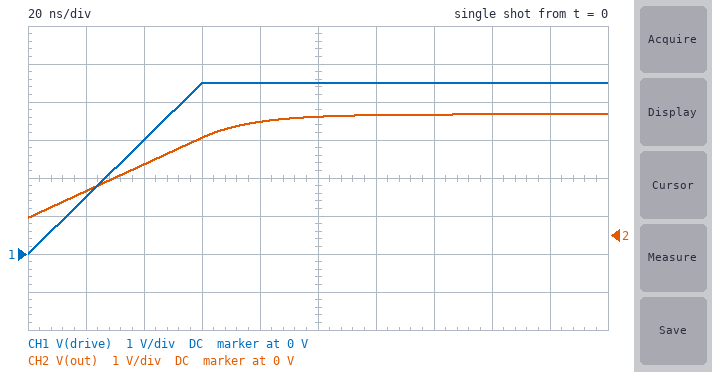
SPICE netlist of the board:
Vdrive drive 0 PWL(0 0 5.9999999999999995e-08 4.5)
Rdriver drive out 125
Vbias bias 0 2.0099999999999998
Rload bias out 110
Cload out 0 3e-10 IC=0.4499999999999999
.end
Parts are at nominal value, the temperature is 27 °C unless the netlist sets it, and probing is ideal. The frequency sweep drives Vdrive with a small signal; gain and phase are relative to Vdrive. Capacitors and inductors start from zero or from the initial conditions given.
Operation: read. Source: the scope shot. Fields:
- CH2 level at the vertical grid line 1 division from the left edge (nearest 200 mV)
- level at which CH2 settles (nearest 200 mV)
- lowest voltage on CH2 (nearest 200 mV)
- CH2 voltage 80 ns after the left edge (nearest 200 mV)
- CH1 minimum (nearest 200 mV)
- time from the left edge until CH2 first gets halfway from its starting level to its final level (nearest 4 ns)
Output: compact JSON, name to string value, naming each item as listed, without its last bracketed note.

{"CH2 level at the vertical grid line 1 division from the left edge": "1.2 V", "level at which CH2 settles": "3.2 V", "lowest voltage on CH2": "400 mV", "CH2 voltage 80 ns after the left edge": "3.0 V", "CH1 minimum": "0 V", "time from the left edge until CH2 first gets halfway from its starting level to its final level": "40 ns"}
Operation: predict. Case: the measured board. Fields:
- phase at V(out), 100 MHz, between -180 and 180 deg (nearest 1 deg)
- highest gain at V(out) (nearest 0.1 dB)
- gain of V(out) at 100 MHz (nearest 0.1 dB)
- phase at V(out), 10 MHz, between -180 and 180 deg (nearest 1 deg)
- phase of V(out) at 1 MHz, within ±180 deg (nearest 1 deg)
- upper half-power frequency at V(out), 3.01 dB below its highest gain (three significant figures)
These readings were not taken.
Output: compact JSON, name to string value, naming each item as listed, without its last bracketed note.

{"phase at V(out), 100 MHz, between -180 and 180 deg": "-85 deg", "highest gain at V(out)": "-6.6 dB", "gain of V(out) at 100 MHz": "-27.5 dB", "phase at V(out), 10 MHz, between -180 and 180 deg": "-48 deg", "phase of V(out) at 1 MHz, within ±180 deg": "-6 deg", "upper half-power frequency at V(out), 3.01 dB below its highest gain": "9.07 MHz"}
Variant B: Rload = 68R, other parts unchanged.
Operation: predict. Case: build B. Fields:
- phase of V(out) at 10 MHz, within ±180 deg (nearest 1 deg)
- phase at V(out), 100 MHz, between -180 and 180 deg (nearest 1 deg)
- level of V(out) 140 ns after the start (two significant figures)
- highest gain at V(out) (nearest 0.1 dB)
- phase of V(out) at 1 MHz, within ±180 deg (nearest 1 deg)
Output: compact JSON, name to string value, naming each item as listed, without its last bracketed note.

{"phase of V(out) at 10 MHz, within ±180 deg": "-40 deg", "phase at V(out), 100 MHz, between -180 and 180 deg": "-83 deg", "level of V(out) 140 ns after the start": "2.9 V", "highest gain at V(out)": "-9.1 dB", "phase of V(out) at 1 MHz, within ±180 deg": "-5 deg"}
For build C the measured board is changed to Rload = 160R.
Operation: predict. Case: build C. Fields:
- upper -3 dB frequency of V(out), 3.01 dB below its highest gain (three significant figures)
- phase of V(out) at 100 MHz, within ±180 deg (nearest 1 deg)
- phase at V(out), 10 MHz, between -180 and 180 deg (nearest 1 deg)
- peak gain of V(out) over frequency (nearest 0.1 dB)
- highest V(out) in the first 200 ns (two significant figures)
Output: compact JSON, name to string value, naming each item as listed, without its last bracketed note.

{"upper -3 dB frequency of V(out), 3.01 dB below its highest gain": "7.56 MHz", "phase of V(out) at 100 MHz, within ±180 deg": "-86 deg", "phase at V(out), 10 MHz, between -180 and 180 deg": "-53 deg", "peak gain of V(out) over frequency": "-5.0 dB", "highest V(out) in the first 200 ns": "3.4 V"}
